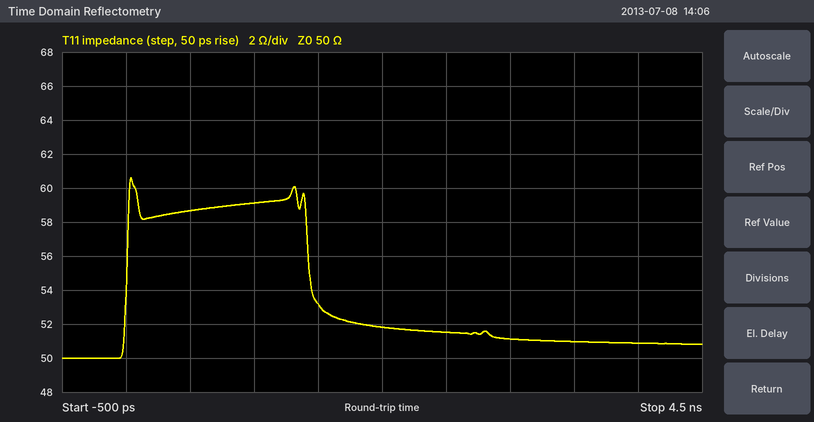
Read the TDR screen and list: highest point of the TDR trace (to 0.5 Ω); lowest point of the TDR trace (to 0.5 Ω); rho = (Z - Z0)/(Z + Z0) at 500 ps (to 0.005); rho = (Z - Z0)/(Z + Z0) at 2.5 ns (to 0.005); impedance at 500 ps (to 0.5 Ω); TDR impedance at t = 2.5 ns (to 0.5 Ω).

60.5 Ω
50.0 Ω
+0.080
+0.015
58.5 Ω
51.5 Ω
